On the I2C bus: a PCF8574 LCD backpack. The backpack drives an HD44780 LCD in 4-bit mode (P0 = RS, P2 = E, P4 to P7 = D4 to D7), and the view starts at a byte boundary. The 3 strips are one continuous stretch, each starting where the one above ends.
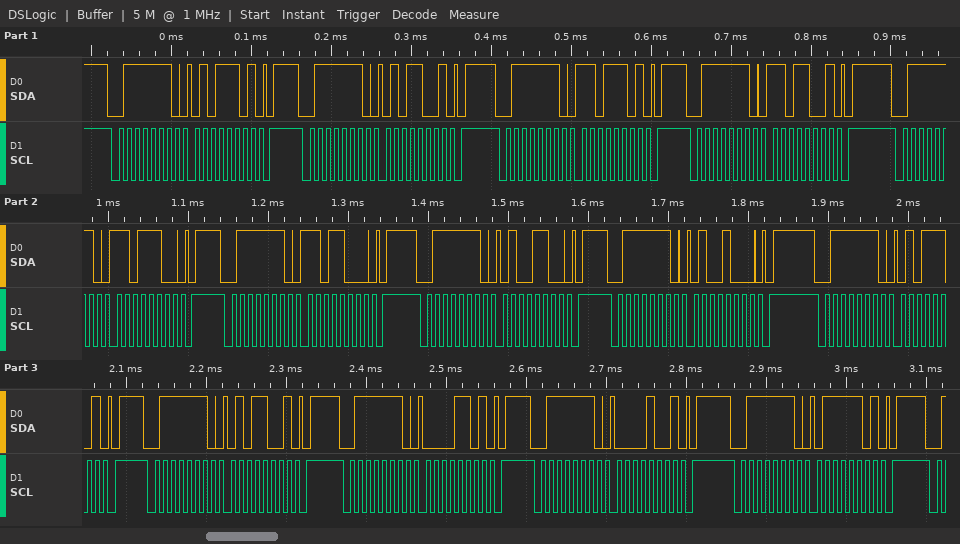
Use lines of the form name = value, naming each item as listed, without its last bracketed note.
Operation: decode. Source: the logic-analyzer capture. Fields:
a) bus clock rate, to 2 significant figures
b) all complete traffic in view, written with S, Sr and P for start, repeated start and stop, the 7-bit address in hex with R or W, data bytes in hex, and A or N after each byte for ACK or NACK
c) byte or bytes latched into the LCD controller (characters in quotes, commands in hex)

bus clock rate, to 2 significant figures = 100 kHz
all complete traffic in view, written with S, Sr and P for start, repeated start and stop, the 7-bit address in hex with R or W, data bytes in hex, and A or N after each byte for ACK or NACK = S 3FW A 5D A P S 3FW A 59 A P S 3FW A DD A P S 3FW A D9 A P S 3FW A DC A P S 3FW A D8 A P S 3FW A 4C A P S 3FW A 48 A P S 3FW A 5D A P S 3FW A 59 A P S 3FW A 0D A P S 3FW A 09 A P S 3FW A 7D A P
byte or bytes latched into the LCD controller = ']' 0xD4 'P'
